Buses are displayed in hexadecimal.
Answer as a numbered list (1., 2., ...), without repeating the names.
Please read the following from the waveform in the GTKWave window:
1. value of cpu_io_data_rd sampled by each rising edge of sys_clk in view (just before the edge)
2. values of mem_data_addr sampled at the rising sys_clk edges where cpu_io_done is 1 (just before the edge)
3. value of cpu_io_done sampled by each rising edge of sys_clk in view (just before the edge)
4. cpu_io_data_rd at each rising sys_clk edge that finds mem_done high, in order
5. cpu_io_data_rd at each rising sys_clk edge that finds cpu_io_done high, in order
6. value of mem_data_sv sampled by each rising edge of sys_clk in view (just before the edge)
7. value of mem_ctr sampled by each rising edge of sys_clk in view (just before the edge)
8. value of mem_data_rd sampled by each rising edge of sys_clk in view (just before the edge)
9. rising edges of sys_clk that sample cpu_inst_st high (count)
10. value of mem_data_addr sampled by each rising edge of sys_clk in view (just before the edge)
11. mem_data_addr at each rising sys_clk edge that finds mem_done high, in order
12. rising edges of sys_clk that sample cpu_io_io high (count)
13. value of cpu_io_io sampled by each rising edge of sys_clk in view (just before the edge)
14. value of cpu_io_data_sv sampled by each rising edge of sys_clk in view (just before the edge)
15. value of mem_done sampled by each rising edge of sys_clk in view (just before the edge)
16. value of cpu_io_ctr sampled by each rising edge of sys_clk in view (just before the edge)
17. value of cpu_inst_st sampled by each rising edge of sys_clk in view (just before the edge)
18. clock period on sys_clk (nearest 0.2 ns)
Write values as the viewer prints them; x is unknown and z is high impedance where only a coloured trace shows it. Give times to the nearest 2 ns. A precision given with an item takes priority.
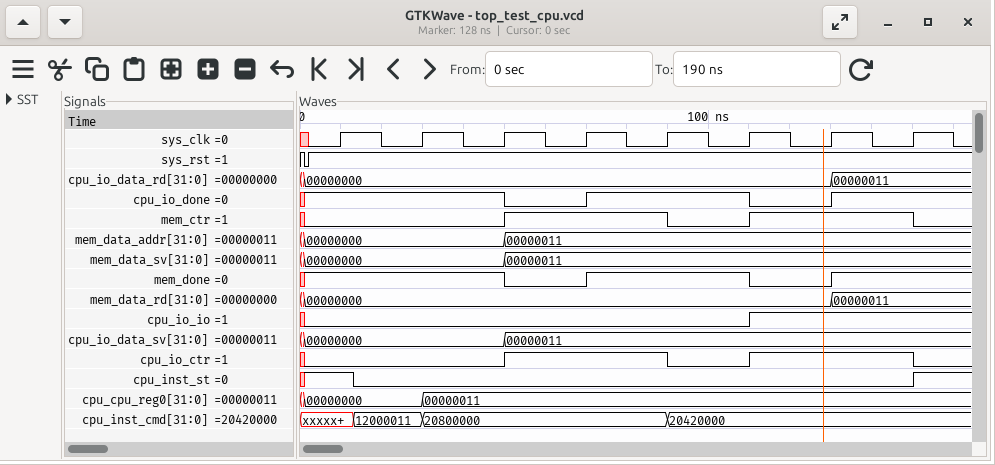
1. 00000000, 00000000, 00000000, 00000000, 00000000, 00000000, 00000000, 00000011
2. 00000000, 00000000, 00000000, 00000011, 00000011, 00000011
3. 1 1 1 0 1 1 0 1
4. 00000000, 00000000, 00000000, 00000000, 00000000, 00000011
5. 00000000, 00000000, 00000000, 00000000, 00000000, 00000011
6. 00000000, 00000000, 00000000, 00000011, 00000011, 00000011, 00000011, 00000011
7. 0 0 0 1 1 0 1 1
8. 00000000, 00000000, 00000000, 00000000, 00000000, 00000000, 00000000, 00000011
9. 1
10. 00000000, 00000000, 00000000, 00000011, 00000011, 00000011, 00000011, 00000011
11. 00000000, 00000000, 00000000, 00000011, 00000011, 00000011
12. 2
13. 0 0 0 0 0 0 1 1
14. 00000000, 00000000, 00000000, 00000011, 00000011, 00000011, 00000011, 00000011
15. 1 1 1 0 1 1 0 1
16. 0 0 0 1 1 0 1 1
17. 1 0 0 0 0 0 0 0
18. 20 ns
